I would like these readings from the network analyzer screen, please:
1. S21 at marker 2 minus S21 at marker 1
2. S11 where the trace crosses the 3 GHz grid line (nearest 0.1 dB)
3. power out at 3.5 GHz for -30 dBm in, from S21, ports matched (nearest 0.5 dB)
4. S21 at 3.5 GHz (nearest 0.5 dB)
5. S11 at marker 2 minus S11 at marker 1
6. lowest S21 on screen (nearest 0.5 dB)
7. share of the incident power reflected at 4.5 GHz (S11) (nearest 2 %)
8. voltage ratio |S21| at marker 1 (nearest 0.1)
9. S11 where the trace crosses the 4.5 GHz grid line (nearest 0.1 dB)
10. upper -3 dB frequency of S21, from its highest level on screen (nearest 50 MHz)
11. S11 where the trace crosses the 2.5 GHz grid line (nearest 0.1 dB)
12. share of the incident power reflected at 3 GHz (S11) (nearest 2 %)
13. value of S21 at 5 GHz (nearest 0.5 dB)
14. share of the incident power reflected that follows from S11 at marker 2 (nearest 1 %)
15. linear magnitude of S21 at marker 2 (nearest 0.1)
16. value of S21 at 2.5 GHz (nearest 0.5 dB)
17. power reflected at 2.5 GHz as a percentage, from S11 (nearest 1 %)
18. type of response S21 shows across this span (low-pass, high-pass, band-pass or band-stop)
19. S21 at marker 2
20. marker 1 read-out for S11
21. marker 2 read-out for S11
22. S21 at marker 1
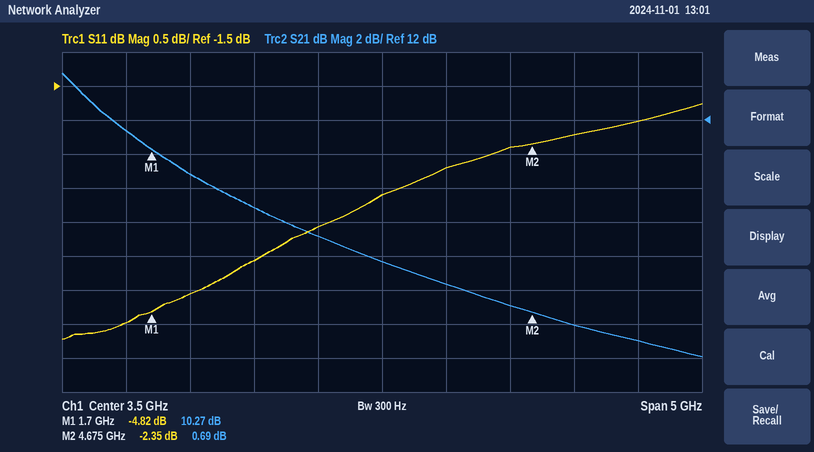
-9.58 dB
-3.6 dB
-26.5 dBm
3.5 dB
2.47 dB
-2.0 dB
58 %
3.3
-2.4 dB
1.45 GHz
-4.1 dB
44 %
0.0 dB
58 %
1.1
7.0 dB
39 %
low-pass
0.69 dB
-4.82 dB
-2.35 dB
10.27 dB
